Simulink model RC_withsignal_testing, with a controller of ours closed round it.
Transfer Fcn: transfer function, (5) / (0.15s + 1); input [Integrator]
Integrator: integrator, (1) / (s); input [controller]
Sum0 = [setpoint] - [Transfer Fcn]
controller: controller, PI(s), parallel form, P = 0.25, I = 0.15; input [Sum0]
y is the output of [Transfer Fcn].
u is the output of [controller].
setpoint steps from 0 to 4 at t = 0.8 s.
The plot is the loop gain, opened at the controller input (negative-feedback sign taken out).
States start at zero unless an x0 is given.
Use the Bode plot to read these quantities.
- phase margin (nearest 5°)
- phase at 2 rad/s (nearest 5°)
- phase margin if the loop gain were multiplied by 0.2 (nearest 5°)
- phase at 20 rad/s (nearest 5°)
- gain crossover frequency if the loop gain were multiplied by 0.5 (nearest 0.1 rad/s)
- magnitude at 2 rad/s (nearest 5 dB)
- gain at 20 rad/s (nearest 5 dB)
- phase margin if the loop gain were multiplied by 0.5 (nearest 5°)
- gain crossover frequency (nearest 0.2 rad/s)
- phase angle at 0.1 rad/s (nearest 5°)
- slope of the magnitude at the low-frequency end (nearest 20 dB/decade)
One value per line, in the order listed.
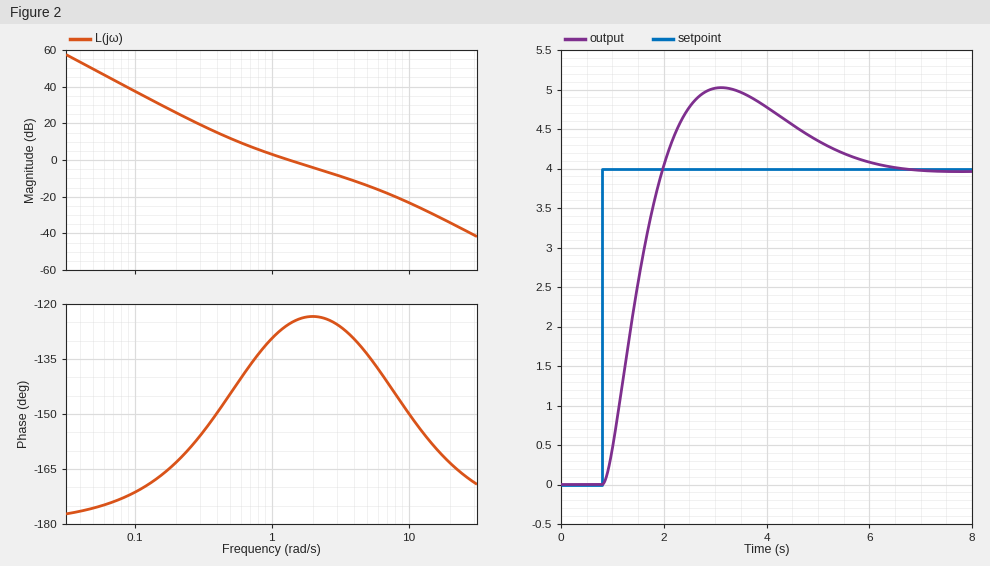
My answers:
55°
-125°
30°
-165°
0.8 rad/s
-5 dB
-35 dB
45°
1.4 rad/s
-170°
-40 dB/decade
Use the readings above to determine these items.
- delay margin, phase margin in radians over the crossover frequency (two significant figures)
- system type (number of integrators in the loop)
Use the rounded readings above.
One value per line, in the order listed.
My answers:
0.69 s
2
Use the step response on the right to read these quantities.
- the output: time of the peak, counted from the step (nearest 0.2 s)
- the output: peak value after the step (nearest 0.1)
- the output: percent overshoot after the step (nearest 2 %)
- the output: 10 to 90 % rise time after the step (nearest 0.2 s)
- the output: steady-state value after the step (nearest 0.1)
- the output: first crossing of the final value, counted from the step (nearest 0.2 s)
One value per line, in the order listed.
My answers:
2.4 s
5.0
26 %
0.8 s
4.0
1.2 s
